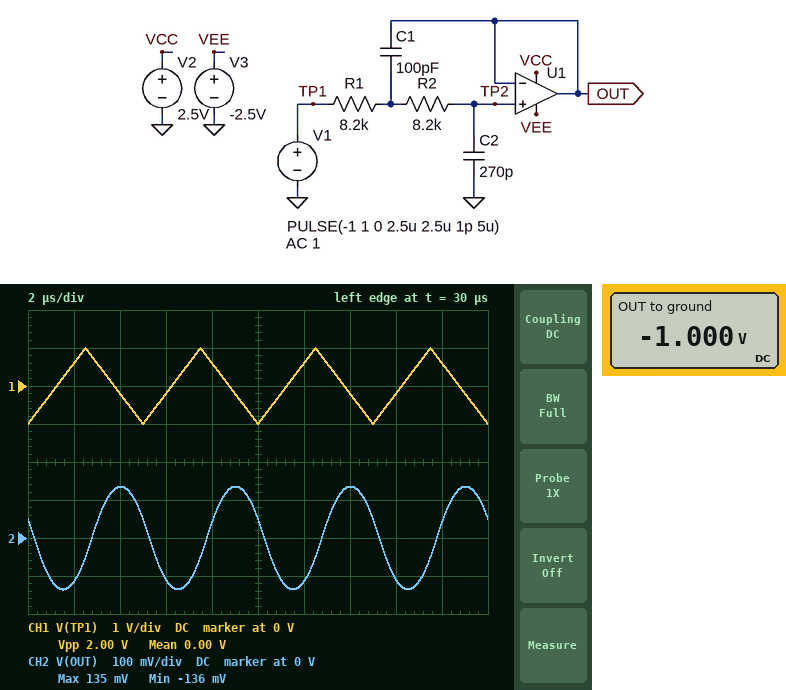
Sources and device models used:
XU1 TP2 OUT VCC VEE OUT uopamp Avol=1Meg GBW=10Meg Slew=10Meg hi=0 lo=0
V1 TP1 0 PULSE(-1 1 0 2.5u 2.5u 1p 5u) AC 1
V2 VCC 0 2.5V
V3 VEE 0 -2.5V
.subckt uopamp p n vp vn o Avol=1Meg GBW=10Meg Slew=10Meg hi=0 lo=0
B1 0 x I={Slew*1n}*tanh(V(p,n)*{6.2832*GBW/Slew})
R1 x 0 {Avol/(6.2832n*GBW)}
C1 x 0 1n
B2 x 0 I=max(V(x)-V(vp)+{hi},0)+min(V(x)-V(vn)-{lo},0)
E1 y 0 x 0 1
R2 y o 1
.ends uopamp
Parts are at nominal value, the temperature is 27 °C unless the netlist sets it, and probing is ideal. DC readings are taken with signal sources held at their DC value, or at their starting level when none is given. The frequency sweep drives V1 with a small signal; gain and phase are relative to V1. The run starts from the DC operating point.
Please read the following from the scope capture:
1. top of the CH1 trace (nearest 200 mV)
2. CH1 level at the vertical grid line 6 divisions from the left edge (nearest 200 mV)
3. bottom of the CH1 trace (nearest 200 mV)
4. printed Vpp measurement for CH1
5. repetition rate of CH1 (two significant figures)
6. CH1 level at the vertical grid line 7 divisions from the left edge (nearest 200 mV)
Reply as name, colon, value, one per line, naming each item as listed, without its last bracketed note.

top of the CH1 trace: 1.0 V
CH1 level at the vertical grid line 6 divisions from the left edge: 600 mV
bottom of the CH1 trace: -1.0 V
printed Vpp measurement for CH1: 2.00 V
repetition rate of CH1: 200 kHz
CH1 level at the vertical grid line 7 divisions from the left edge: -200 mV
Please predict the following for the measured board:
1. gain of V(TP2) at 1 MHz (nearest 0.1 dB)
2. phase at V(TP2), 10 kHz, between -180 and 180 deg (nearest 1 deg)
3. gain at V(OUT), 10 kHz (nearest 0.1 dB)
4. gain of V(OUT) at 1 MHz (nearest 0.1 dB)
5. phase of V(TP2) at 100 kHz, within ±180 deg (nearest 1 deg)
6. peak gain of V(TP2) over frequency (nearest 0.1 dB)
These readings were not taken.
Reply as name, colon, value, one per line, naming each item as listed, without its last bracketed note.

gain of V(TP2) at 1 MHz: -37.7 dB
phase at V(TP2), 10 kHz, between -180 and 180 deg: -16 deg
gain at V(OUT), 10 kHz: -0.3 dB
gain of V(OUT) at 1 MHz: -37.7 dB
phase of V(TP2) at 100 kHz, within ±180 deg: -84 deg
peak gain of V(TP2) over frequency: 0 dB
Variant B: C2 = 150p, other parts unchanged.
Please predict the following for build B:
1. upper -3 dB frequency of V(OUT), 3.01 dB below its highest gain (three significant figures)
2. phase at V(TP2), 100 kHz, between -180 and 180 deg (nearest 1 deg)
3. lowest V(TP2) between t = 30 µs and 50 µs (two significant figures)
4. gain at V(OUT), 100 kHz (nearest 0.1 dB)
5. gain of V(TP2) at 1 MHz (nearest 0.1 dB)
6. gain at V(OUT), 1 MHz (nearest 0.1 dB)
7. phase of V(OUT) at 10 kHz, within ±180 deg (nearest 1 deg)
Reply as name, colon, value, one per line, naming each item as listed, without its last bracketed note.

upper -3 dB frequency of V(OUT), 3.01 dB below its highest gain: 77.2 kHz
phase at V(TP2), 100 kHz, between -180 and 180 deg: -69 deg
lowest V(TP2) between t = 30 µs and 50 µs: -250 mV
gain at V(OUT), 100 kHz: -4.4 dB
gain of V(TP2) at 1 MHz: -32.5 dB
gain at V(OUT), 1 MHz: -32.6 dB
phase of V(OUT) at 10 kHz, within ±180 deg: -9 deg
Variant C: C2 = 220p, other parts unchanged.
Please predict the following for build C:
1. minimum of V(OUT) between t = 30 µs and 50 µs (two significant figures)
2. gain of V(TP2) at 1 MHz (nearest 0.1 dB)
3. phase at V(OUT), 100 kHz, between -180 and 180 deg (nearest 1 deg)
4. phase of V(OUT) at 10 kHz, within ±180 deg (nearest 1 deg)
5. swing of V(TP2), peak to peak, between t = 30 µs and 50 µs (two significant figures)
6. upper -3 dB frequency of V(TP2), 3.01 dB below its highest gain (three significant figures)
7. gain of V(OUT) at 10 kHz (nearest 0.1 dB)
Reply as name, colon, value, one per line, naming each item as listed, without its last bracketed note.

minimum of V(OUT) between t = 30 µs and 50 µs: -170 mV
gain of V(TP2) at 1 MHz: -35.9 dB
phase at V(OUT), 100 kHz, between -180 and 180 deg: -80 deg
phase of V(OUT) at 10 kHz, within ±180 deg: -13 deg
swing of V(TP2), peak to peak, between t = 30 µs and 50 µs: 340 mV
upper -3 dB frequency of V(TP2), 3.01 dB below its highest gain: 49.7 kHz
gain of V(OUT) at 10 kHz: -0.2 dB
